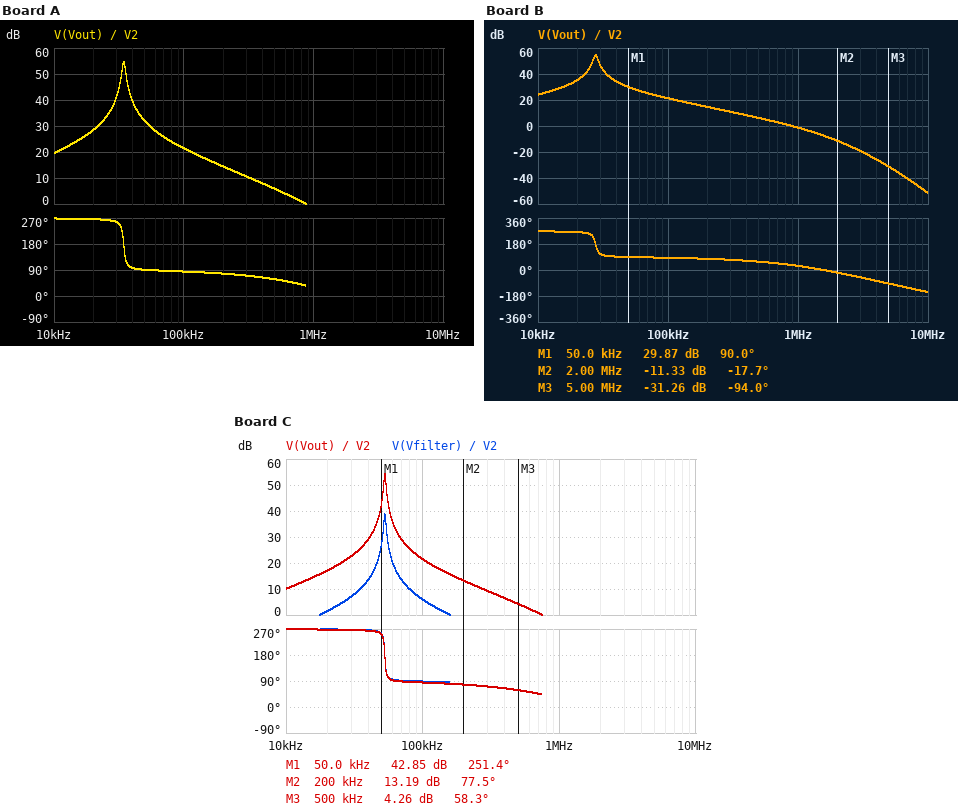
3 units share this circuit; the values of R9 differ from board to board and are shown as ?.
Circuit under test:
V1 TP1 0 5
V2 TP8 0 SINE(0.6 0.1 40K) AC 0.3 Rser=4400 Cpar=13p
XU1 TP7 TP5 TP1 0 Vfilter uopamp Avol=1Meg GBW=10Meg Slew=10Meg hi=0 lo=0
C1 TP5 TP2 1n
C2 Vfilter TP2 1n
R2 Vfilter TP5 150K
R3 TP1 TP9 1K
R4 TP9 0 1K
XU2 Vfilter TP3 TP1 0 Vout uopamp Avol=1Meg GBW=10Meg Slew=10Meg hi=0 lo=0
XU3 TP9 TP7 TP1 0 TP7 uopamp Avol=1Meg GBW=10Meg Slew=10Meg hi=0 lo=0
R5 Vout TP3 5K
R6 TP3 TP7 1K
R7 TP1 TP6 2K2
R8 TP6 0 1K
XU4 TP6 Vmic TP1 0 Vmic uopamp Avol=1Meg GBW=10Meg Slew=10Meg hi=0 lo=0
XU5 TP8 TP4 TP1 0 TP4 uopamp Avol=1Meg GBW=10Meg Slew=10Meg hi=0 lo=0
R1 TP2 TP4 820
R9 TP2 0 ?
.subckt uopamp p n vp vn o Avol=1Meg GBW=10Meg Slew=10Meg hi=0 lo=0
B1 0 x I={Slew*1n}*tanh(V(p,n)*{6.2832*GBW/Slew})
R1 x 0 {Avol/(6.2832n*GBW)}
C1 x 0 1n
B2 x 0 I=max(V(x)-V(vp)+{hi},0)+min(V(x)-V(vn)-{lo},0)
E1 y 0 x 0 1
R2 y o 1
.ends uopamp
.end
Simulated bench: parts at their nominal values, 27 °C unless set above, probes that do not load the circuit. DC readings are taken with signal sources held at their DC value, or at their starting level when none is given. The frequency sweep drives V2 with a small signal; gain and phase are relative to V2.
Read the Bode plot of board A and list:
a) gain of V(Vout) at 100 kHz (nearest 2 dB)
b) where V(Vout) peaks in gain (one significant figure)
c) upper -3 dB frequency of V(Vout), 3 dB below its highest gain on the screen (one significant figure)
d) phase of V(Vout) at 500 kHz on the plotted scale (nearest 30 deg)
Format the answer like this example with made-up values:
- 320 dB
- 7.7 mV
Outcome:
- 22 dB
- 30 kHz
- 40 kHz
- 60 deg
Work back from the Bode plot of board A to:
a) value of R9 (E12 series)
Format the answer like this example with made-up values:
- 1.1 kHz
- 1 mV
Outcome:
- 150 Ω
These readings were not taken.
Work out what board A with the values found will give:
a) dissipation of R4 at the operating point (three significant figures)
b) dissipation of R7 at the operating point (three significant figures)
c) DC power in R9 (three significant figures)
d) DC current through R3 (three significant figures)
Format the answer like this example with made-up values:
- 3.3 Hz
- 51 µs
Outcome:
- 6.25 mW
- 5.37 mW
- 57.4 µW
- 2.50 mA
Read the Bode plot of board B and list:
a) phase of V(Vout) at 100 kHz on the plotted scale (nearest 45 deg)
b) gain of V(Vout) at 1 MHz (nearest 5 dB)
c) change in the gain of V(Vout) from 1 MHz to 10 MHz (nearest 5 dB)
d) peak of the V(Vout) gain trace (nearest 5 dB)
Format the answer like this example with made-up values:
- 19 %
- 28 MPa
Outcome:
- 90 deg
- 0 dB
- -50 dB
- 55 dB
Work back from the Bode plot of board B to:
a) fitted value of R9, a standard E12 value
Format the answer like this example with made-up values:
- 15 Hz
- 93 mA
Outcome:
- 270 Ω
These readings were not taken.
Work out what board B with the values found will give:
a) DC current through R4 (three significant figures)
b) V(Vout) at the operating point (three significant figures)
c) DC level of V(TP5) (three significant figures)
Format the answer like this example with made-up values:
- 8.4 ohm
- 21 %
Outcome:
- 2.50 mA
- 2.50 V
- 2.50 V
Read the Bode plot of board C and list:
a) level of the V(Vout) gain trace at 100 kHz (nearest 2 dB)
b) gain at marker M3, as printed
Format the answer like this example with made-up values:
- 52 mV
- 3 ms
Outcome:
- 22 dB
- 4.26 dB
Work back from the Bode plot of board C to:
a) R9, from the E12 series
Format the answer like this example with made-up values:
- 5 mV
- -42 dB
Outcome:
- 47 Ω
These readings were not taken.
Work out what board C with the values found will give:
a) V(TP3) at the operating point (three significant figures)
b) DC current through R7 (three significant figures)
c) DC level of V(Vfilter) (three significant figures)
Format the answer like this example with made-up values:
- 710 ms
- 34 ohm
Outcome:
- 2.50 V
- 1.56 mA
- 2.50 V
